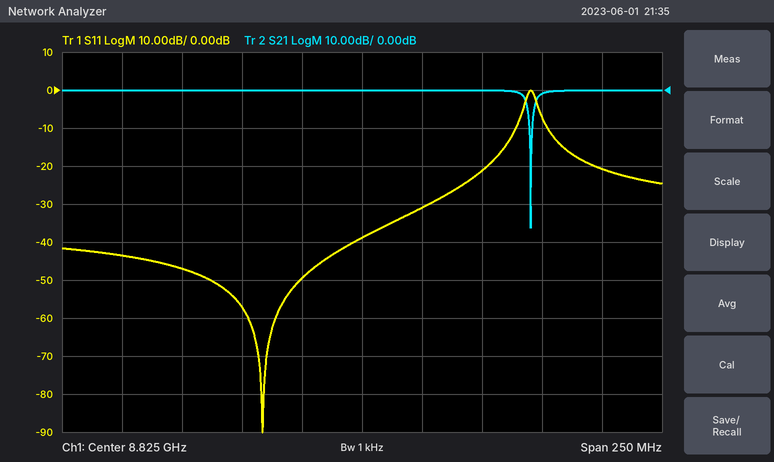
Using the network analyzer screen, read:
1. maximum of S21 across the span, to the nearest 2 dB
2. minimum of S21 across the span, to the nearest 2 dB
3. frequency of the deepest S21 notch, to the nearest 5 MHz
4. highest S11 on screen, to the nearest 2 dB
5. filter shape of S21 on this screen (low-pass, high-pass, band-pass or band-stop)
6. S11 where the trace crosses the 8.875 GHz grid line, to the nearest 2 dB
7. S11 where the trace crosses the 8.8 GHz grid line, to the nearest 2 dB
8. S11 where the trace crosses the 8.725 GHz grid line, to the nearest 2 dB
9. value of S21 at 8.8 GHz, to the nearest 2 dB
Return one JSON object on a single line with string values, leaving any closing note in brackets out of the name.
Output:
{"maximum of S21 across the span, to the nearest 2 dB": "0 dB", "minimum of S21 across the span, to the nearest 2 dB": "-36 dB", "frequency of the deepest S21 notch, to the nearest 5 MHz": "8.895 GHz", "highest S11 on screen, to the nearest 2 dB": "0 dB", "filter shape of S21 on this screen": "band-stop", "S11 where the trace crosses the 8.875 GHz grid line, to the nearest 2 dB": "-22 dB", "S11 where the trace crosses the 8.8 GHz grid line, to the nearest 2 dB": "-50 dB", "S11 where the trace crosses the 8.725 GHz grid line, to the nearest 2 dB": "-44 dB", "value of S21 at 8.8 GHz, to the nearest 2 dB": "0 dB"}
